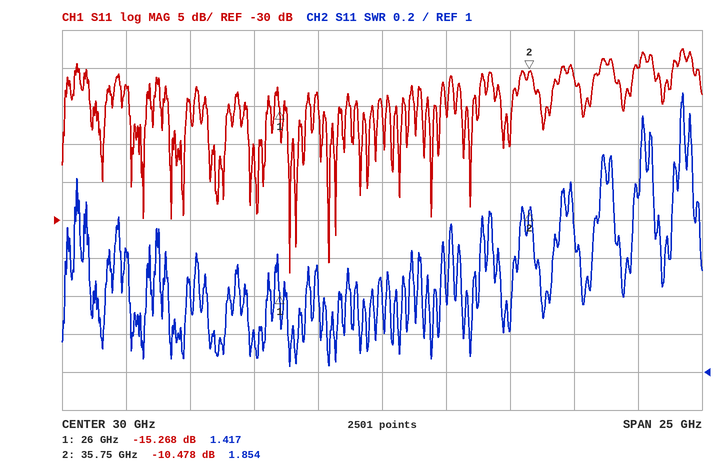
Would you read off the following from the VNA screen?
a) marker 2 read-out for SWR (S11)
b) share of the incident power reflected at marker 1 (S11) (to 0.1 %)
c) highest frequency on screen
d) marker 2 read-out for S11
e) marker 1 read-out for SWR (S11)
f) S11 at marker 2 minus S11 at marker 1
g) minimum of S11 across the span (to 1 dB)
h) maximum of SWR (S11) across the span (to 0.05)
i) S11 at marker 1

1.854
3.0 %
42.5 GHz
-10.478 dB
1.417
4.790 dB
-37 dB
2.45
-15.268 dB
